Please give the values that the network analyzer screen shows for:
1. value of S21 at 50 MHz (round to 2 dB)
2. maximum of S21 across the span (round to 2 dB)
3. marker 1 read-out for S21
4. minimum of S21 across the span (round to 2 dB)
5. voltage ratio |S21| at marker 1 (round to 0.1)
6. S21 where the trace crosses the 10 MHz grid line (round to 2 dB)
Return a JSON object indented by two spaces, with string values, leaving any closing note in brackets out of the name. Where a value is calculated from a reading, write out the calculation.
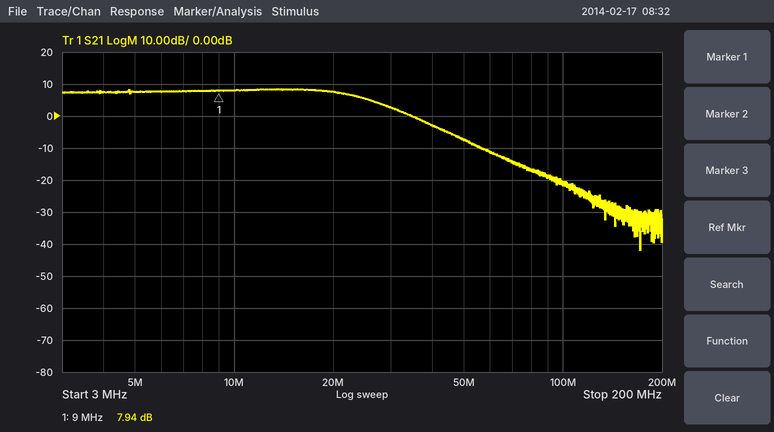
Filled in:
{
  "value of S21 at 50 MHz": "-8 dB",
  "maximum of S21 across the span": "8 dB",
  "marker 1 read-out for S21": "7.94 dB",
  "minimum of S21 across the span": "-42 dB",
  "voltage ratio |S21| at marker 1": "10^(7.94/20) ≈ 2.5",
  "S21 where the trace crosses the 10 MHz grid line": "8 dB"
}
